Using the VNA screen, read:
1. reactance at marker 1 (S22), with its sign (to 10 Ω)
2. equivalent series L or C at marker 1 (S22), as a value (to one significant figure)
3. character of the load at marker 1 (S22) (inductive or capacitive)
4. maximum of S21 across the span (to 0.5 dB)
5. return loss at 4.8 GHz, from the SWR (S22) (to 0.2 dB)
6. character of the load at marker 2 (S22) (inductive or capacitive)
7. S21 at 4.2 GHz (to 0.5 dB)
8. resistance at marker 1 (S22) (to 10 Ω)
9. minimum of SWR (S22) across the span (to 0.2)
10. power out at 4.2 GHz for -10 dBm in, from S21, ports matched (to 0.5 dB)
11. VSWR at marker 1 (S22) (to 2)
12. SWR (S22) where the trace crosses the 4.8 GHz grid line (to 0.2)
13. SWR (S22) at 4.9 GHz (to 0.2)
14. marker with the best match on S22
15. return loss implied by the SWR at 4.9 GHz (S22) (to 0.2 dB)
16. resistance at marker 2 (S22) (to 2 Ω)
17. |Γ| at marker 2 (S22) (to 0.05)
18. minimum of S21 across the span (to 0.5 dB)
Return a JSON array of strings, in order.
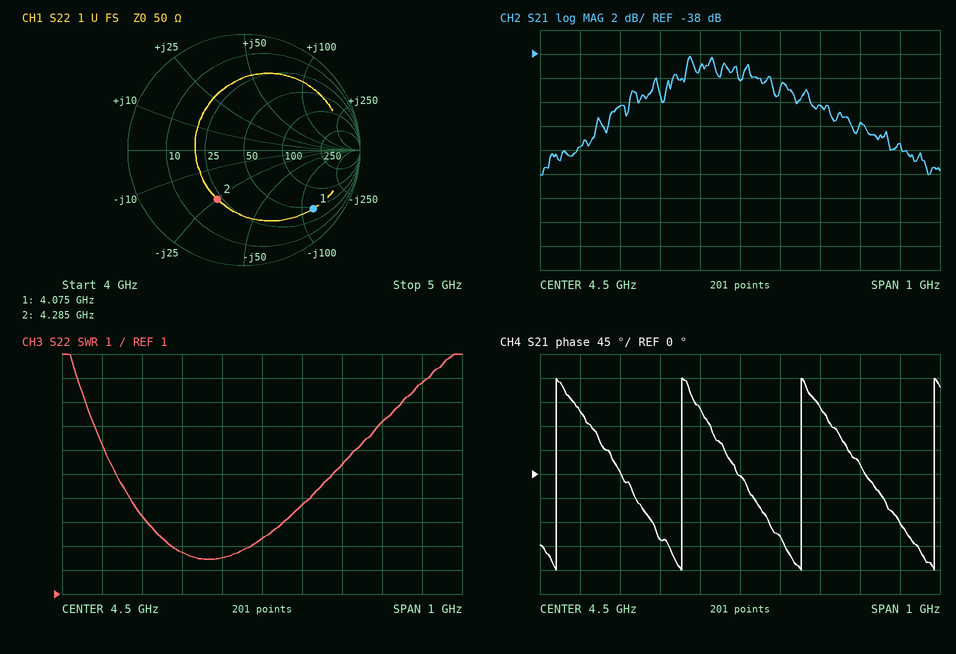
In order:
["-120 Ω", "300 fF", "capacitive", "-38.0 dB", "2.2 dB", "capacitive", "-42.5 dB", "50 Ω", "2.4", "-52.5 dBm", "8", "8.2", "9.8", "marker 2", "1.8 dB", "22 Ω", "0.50", "-48.0 dB"]
